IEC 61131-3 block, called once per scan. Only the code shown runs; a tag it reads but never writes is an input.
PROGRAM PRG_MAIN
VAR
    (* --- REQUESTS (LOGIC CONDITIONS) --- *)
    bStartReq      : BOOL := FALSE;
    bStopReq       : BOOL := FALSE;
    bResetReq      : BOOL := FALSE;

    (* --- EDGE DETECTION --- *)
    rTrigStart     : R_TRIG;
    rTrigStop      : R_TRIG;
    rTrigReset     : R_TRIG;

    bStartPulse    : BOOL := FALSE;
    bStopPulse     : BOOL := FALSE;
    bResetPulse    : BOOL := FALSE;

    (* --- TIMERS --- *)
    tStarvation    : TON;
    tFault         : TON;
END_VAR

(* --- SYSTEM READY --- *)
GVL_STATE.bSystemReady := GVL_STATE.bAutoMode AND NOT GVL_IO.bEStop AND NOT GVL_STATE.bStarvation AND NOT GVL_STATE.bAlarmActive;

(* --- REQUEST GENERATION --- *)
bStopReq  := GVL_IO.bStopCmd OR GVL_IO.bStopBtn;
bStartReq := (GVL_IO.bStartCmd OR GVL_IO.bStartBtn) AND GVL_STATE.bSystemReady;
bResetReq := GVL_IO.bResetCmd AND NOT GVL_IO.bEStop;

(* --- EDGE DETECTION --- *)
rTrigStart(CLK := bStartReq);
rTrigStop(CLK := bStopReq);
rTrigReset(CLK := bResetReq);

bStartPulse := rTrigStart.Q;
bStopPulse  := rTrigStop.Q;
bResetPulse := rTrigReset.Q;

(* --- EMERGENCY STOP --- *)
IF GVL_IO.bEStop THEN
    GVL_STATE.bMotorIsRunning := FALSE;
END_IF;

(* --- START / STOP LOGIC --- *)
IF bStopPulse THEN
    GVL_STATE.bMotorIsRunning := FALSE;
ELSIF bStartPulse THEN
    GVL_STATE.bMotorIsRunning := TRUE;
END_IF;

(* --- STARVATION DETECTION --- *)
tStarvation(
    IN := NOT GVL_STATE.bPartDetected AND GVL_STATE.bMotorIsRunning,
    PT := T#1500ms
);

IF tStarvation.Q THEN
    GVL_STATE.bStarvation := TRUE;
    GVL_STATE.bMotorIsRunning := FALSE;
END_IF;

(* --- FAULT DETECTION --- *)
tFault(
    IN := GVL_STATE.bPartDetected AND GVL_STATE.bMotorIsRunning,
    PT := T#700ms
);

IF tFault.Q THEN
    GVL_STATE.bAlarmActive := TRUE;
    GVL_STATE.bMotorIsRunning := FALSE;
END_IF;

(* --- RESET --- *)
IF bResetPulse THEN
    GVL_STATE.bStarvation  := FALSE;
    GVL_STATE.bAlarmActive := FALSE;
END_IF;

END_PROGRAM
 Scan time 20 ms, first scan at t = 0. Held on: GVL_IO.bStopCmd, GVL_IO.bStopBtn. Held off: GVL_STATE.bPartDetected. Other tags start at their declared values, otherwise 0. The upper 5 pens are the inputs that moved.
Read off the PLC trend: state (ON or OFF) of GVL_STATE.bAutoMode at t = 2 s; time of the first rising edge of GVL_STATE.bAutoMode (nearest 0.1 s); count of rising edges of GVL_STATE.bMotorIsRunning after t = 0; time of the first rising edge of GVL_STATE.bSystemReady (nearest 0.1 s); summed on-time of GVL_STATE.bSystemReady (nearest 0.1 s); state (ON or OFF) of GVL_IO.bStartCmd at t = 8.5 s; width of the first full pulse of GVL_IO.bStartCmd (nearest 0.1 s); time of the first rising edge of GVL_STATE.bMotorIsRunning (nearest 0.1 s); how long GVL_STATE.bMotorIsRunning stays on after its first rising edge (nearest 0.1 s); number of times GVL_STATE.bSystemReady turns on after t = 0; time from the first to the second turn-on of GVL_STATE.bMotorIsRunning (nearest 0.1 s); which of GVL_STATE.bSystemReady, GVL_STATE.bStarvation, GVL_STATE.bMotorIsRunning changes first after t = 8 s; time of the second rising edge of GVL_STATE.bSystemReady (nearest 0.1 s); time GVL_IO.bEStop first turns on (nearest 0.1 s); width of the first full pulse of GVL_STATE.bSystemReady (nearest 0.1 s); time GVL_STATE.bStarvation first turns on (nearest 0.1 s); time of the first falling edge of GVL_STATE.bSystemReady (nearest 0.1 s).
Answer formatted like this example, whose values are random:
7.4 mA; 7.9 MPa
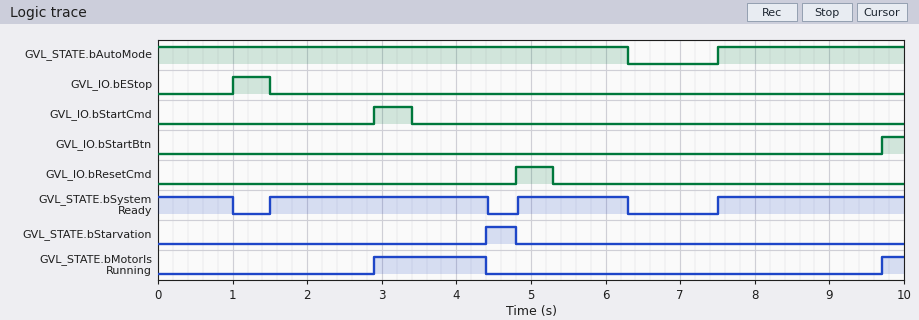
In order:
ON; 7.5 s; 2; 1.5 s; 7.9 s; OFF; 0.5 s; 2.9 s; 1.5 s; 3; 6.8 s; GVL_STATE.bMotorIsRunning; 4.8 s; 1.0 s; 2.9 s; 4.4 s; 1.0 s
